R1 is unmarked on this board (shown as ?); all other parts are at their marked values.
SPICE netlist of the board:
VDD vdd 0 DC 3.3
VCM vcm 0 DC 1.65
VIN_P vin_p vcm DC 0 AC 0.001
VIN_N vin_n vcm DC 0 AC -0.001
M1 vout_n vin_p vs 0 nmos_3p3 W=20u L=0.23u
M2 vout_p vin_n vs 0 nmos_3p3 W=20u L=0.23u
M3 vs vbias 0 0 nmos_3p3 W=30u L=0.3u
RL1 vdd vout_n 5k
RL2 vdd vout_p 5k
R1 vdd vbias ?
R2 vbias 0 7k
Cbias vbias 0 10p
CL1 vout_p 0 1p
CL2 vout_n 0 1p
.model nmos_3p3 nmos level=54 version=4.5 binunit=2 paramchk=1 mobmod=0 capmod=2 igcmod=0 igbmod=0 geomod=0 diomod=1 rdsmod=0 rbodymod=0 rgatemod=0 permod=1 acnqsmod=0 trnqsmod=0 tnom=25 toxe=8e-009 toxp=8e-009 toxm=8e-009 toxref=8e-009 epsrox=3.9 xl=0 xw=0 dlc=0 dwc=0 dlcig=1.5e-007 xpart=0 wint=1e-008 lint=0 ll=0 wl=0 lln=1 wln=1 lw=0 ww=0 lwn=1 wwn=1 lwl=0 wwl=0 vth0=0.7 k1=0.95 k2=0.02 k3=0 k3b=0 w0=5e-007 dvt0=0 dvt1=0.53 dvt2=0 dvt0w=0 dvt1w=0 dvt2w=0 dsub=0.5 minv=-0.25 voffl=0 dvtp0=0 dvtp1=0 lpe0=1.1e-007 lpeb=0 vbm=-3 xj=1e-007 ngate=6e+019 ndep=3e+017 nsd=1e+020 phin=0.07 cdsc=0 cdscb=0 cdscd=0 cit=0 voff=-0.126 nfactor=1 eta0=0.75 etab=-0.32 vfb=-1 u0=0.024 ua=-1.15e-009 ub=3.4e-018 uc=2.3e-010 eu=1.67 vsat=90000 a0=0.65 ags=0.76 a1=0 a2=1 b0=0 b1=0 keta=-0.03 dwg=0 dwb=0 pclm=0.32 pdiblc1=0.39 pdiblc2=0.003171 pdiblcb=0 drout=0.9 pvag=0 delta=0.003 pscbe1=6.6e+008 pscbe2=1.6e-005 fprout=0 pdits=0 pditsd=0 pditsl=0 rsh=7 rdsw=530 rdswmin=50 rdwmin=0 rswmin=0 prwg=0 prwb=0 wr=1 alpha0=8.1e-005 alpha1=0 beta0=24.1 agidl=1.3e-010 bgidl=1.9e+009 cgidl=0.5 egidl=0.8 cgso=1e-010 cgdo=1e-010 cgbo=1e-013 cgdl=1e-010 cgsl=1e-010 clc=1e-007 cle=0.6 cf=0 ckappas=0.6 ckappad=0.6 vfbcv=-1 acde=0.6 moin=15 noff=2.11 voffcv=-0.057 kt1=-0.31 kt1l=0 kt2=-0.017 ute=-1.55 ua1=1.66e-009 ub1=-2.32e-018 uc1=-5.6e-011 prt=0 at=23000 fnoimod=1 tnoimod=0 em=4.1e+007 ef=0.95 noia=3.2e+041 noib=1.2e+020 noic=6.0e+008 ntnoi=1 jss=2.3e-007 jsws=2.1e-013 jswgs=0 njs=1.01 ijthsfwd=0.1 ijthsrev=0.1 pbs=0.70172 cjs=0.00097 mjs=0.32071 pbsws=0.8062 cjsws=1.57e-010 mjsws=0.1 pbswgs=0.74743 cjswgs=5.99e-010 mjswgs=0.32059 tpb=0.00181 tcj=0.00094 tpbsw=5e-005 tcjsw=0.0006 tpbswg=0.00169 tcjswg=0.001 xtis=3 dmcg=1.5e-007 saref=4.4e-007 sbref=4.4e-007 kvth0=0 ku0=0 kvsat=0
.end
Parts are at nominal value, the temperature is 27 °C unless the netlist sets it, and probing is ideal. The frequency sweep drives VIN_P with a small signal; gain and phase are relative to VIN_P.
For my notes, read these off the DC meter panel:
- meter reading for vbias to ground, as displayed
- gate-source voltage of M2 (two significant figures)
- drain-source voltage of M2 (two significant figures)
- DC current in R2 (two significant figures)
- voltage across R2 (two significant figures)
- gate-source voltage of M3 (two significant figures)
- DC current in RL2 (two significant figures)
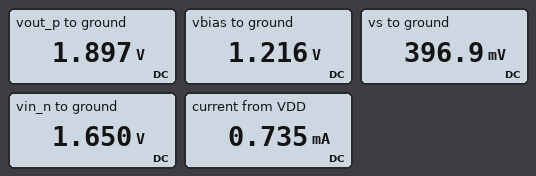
1.216 V
1.3 V
1.5 V
170 µA
1.2 V
1.2 V
280 µA
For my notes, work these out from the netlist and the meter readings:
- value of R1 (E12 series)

12 kΩ
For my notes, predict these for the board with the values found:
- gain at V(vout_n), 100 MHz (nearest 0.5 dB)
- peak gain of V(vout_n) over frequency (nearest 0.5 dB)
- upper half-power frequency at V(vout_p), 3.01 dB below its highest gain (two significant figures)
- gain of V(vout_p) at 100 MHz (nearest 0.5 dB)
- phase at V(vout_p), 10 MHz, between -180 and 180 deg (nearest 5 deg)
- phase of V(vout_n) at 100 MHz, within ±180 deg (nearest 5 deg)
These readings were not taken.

2.5 dB
9.5 dB
50 MHz
1.5 dB
-10 deg
115 deg
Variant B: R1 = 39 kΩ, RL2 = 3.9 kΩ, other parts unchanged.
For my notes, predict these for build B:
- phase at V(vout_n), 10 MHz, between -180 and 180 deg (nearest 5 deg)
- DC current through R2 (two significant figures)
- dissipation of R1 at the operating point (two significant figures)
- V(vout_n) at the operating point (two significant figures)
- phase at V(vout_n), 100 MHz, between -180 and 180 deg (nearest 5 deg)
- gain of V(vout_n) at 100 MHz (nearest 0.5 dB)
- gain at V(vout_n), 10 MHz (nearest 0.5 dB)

105 deg
72 µA
200 µW
3.3 V
20 deg
-52.0 dB
-60.5 dB
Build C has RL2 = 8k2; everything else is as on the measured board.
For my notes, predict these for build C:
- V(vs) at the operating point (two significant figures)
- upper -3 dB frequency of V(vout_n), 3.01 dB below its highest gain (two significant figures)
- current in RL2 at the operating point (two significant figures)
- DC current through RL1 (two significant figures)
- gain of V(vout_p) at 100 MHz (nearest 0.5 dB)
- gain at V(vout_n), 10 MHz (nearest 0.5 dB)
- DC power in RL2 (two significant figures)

380 mV
58 MHz
250 µA
310 µA
2.0 dB
8.5 dB
510 µW
